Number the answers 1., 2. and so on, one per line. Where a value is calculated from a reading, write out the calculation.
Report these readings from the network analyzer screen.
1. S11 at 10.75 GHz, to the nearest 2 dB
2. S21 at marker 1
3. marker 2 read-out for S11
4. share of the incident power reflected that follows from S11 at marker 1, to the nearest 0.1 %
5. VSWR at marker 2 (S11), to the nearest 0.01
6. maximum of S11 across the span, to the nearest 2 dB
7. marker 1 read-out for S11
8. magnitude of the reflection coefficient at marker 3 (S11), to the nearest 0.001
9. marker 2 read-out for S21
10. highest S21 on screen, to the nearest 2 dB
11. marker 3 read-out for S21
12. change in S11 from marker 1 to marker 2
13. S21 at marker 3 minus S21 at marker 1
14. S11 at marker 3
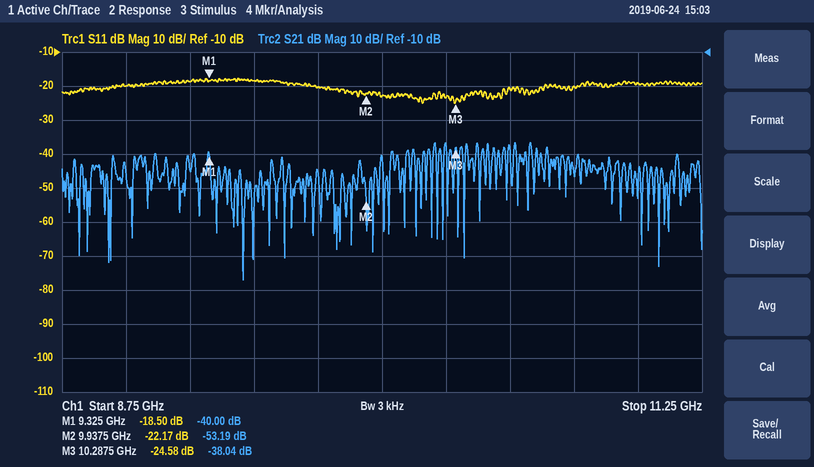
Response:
1. -20 dB
2. -40.00 dB
3. -22.17 dB
4. 10^(-18.5/10) ≈ 1.4 %
5. (1 + 0.0779)/(1 − 0.0779) ≈ 1.17
6. -18 dB
7. -18.50 dB
8. 10^(-24.58/20) ≈ 0.059
9. -53.19 dB
10. -36 dB
11. -38.04 dB
12. -22.17 − (-18.5) = -3.67 dB
13. -38.04 − (-40) = 1.96 dB
14. -24.58 dB
